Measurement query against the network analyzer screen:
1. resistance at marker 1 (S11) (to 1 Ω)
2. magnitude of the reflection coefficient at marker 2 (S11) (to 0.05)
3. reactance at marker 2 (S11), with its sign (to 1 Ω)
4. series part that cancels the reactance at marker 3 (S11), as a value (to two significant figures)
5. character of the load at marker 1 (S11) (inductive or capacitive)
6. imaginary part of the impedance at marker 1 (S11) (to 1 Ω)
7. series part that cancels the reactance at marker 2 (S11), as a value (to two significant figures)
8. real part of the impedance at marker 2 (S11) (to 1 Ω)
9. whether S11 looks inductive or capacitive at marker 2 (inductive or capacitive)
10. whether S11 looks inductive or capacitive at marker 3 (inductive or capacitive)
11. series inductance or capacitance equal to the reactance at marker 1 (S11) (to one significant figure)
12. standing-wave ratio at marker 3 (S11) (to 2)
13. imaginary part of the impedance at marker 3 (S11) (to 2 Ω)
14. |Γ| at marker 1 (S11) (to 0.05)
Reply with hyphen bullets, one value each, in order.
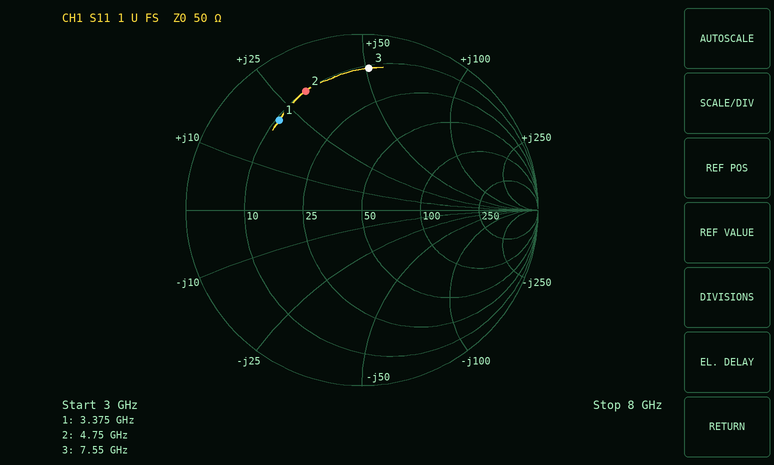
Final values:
- 11 Ω
- 0.75
- +31 Ω
- 410 fF
- inductive
- +21 Ω
- 1.1 pF
- 10 Ω
- inductive
- inductive
- 1.0 nH
- 10
- +52 Ω
- 0.70
